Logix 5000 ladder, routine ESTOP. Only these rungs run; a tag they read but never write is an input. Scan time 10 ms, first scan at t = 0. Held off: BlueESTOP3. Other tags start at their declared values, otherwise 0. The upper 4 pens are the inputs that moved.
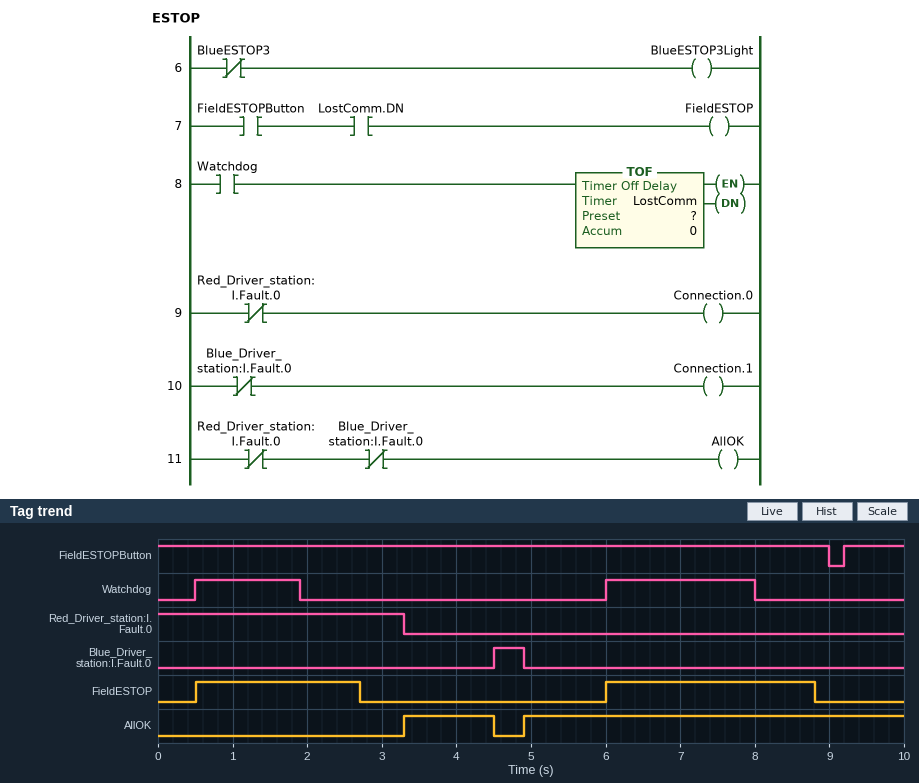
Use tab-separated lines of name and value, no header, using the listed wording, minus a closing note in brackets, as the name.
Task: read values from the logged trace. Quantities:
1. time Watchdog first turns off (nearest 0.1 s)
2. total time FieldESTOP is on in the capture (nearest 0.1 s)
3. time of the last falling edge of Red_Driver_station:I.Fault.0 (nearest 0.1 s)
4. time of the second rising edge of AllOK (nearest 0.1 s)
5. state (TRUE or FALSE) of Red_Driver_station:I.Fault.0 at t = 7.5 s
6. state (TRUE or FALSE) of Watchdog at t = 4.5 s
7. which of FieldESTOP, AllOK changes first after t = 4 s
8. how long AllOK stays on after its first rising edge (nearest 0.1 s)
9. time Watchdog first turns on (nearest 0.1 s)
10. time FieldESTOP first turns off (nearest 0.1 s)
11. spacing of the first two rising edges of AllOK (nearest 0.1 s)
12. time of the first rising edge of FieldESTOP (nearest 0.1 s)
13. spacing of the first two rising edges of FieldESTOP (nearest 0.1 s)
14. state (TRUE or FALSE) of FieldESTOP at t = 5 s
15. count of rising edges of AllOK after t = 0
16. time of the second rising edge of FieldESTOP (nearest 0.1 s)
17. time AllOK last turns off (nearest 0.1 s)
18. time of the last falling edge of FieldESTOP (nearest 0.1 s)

time Watchdog first turns off	1.9 s
total time FieldESTOP is on in the capture	5.0 s
time of the last falling edge of Red_Driver_station:I.Fault.0	3.3 s
time of the second rising edge of AllOK	4.9 s
state (TRUE or FALSE) of Red_Driver_station:I.Fault.0 at t = 7.5 s	FALSE
state (TRUE or FALSE) of Watchdog at t = 4.5 s	FALSE
which of FieldESTOP, AllOK changes first after t = 4 s	AllOK
how long AllOK stays on after its first rising edge	1.2 s
time Watchdog first turns on	0.5 s
time FieldESTOP first turns off	2.7 s
spacing of the first two rising edges of AllOK	1.6 s
time of the first rising edge of FieldESTOP	0.5 s
spacing of the first two rising edges of FieldESTOP	5.5 s
state (TRUE or FALSE) of FieldESTOP at t = 5 s	FALSE
count of rising edges of AllOK after t = 0	2
time of the second rising edge of FieldESTOP	6.0 s
time AllOK last turns off	4.5 s
time of the last falling edge of FieldESTOP	8.8 s
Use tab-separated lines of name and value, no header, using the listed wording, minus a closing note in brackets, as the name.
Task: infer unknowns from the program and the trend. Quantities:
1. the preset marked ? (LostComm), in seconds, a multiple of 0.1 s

the preset marked ? (LostComm), in seconds, a multiple of 0.1 s	0.8 s
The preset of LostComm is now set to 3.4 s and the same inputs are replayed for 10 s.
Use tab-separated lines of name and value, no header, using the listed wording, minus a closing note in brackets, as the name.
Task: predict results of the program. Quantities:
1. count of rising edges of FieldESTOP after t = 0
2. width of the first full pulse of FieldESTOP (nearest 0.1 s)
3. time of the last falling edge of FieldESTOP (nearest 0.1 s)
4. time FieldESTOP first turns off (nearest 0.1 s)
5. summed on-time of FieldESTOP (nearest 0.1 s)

count of rising edges of FieldESTOP after t = 0	3
width of the first full pulse of FieldESTOP	4.8 s
time of the last falling edge of FieldESTOP	9.0 s
time FieldESTOP first turns off	5.3 s
summed on-time of FieldESTOP	8.6 s
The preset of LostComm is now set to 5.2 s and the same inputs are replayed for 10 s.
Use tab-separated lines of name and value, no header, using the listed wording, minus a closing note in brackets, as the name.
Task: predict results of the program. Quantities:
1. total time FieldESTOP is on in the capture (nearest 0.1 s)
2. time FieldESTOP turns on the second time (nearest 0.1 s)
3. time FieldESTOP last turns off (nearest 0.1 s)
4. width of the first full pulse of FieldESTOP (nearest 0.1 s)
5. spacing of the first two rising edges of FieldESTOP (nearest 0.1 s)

total time FieldESTOP is on in the capture	9.3 s
time FieldESTOP turns on the second time	9.2 s
time FieldESTOP last turns off	9.0 s
width of the first full pulse of FieldESTOP	8.5 s
spacing of the first two rising edges of FieldESTOP	8.7 s
